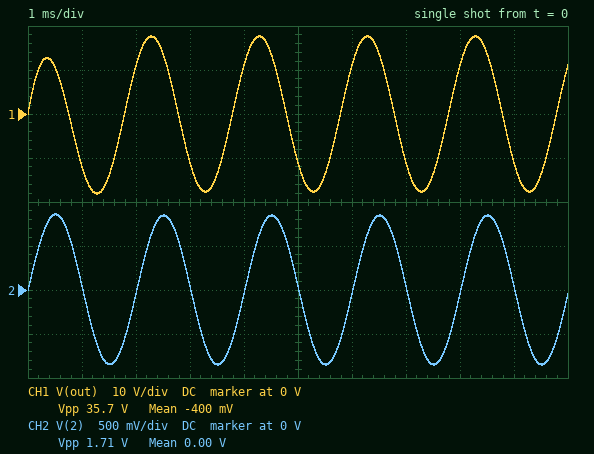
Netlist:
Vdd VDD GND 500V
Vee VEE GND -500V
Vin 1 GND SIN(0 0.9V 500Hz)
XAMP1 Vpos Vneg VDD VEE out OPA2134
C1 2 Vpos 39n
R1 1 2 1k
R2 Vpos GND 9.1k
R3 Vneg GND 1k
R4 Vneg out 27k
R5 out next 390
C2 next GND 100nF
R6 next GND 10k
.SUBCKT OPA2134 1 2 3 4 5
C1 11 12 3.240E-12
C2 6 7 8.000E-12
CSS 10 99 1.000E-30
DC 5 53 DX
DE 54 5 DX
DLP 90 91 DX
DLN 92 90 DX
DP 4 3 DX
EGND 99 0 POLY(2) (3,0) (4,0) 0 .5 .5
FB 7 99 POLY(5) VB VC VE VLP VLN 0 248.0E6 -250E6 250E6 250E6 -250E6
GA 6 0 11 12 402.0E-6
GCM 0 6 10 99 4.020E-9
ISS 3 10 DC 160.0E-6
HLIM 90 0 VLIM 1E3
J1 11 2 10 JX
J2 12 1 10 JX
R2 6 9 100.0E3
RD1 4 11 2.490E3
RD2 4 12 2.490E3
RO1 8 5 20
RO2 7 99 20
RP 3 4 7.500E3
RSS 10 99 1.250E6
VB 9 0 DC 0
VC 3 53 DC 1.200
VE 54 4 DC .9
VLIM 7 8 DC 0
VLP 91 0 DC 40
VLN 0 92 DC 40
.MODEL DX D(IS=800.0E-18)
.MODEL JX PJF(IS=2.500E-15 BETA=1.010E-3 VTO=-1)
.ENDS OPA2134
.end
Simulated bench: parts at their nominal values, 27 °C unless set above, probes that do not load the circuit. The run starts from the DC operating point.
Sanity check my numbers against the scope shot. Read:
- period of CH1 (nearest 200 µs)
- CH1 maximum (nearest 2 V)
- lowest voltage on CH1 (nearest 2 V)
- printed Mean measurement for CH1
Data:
2.0 ms
18 V
-18 V
-400 mV
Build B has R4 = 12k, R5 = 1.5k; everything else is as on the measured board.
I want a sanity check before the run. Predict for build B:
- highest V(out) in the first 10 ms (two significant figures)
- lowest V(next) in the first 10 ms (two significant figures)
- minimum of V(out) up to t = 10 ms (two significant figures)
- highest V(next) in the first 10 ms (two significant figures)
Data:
8.2 V
-6.8 V
-8.4 V
6.6 V
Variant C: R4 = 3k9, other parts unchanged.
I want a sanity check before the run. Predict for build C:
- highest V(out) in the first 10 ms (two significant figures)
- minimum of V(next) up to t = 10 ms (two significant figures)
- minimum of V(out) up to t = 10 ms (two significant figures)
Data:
3.1 V
-3.0 V
-3.2 V
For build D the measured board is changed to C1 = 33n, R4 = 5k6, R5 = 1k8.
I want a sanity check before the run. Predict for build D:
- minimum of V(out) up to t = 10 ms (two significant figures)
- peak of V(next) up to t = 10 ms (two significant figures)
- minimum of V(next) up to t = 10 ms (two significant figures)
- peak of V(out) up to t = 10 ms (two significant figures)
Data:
-3.9 V
3.0 V
-3.0 V
3.9 V
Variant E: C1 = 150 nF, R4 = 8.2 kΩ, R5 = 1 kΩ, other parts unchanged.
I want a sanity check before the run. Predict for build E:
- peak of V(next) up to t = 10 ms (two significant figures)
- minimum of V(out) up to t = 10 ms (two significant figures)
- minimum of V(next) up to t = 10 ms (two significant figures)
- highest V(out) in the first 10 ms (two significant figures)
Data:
6.4 V
-7.9 V
-6.9 V
7.3 V
